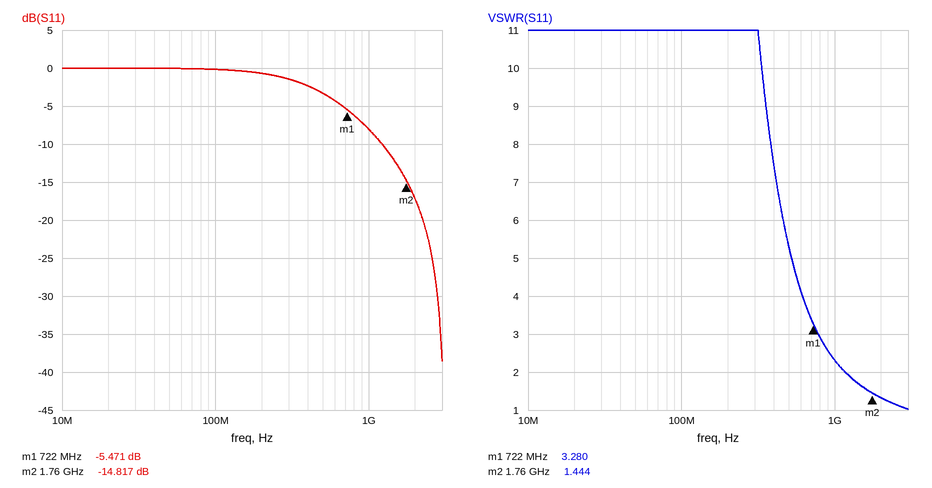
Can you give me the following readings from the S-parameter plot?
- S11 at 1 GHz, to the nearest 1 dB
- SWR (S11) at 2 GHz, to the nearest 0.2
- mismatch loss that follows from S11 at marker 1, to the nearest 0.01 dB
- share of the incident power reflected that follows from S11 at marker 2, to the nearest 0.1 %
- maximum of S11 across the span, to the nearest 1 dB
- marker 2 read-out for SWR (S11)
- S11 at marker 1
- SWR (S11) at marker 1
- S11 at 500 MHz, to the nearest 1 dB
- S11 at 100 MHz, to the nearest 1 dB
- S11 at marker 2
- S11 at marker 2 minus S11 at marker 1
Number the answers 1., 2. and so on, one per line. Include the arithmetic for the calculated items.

1. -8 dB
2. 1.4
3. −10 log10(1 − 10^(-5.471/10)) ≈ 1.45 dB
4. 10^(-14.817/10) ≈ 3.3 %
5. 0 dB
6. 1.444
7. -5.471 dB
8. 3.280
9. -3 dB
10. 0 dB
11. -14.817 dB
12. -14.817 − (-5.471) = -9.346 dB
